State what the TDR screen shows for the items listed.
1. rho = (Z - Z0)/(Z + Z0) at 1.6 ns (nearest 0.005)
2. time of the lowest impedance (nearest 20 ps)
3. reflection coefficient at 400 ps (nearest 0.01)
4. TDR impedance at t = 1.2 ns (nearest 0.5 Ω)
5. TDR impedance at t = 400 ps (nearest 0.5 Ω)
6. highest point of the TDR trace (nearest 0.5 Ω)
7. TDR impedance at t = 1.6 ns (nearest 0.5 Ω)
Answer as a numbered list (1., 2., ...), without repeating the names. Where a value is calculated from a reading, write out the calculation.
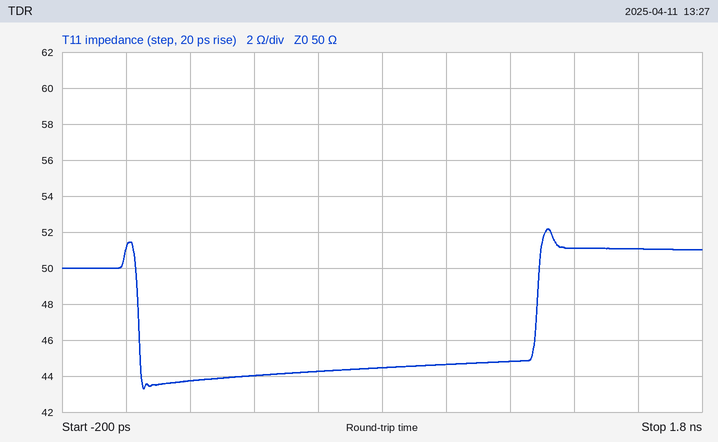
1. (51 − 50)/(51 + 50) ≈ +0.010
2. 60 ps
3. (44 − 50)/(44 + 50) ≈ -0.06
4. 45.0 Ω
5. 44.0 Ω
6. 52.0 Ω
7. 51.0 Ω
